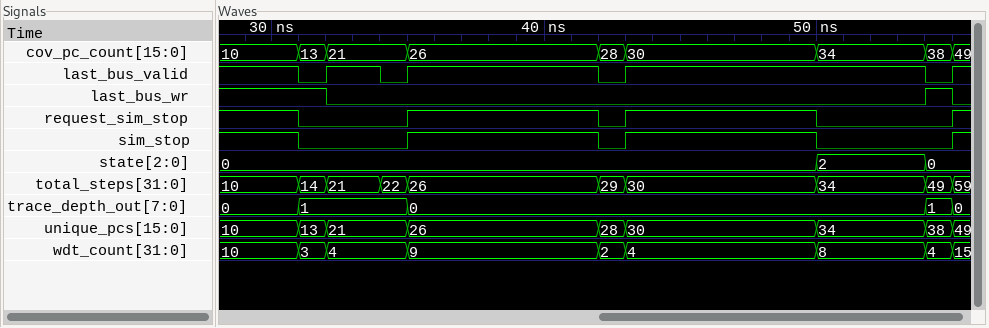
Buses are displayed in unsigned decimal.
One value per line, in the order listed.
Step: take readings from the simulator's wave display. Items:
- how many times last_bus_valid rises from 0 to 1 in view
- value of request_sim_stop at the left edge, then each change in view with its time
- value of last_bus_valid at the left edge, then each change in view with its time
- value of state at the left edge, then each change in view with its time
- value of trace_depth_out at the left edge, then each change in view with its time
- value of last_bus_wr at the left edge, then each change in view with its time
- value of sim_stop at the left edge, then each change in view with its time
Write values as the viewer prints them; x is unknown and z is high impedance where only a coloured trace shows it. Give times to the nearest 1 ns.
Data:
4
1, 0 at 31 ns, 1 at 35 ns, 0 at 42 ns, 1 at 43 ns, 0 at 50 ns, 1 at 55 ns
1, 0 at 31 ns, 1 at 32 ns, 0 at 34 ns, 1 at 35 ns, 0 at 42 ns, 1 at 43 ns, 0 at 54 ns, 1 at 55 ns
0, 2 at 50 ns, 0 at 54 ns
0, 1 at 31 ns, 0 at 35 ns, 1 at 54 ns, 0 at 55 ns
1, 0 at 32 ns, 1 at 54 ns, 0 at 55 ns
1, 0 at 31 ns, 1 at 35 ns, 0 at 42 ns, 1 at 43 ns, 0 at 50 ns, 1 at 55 ns
